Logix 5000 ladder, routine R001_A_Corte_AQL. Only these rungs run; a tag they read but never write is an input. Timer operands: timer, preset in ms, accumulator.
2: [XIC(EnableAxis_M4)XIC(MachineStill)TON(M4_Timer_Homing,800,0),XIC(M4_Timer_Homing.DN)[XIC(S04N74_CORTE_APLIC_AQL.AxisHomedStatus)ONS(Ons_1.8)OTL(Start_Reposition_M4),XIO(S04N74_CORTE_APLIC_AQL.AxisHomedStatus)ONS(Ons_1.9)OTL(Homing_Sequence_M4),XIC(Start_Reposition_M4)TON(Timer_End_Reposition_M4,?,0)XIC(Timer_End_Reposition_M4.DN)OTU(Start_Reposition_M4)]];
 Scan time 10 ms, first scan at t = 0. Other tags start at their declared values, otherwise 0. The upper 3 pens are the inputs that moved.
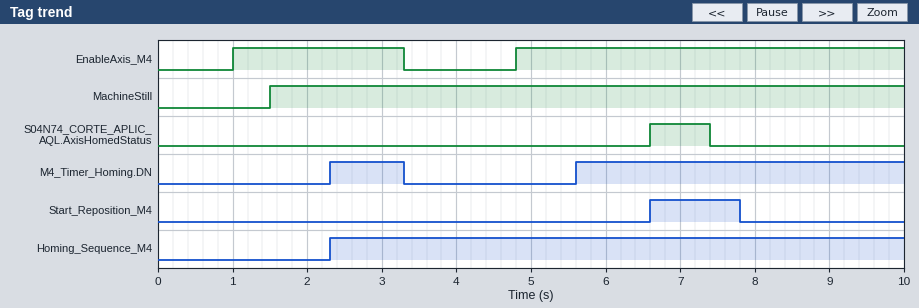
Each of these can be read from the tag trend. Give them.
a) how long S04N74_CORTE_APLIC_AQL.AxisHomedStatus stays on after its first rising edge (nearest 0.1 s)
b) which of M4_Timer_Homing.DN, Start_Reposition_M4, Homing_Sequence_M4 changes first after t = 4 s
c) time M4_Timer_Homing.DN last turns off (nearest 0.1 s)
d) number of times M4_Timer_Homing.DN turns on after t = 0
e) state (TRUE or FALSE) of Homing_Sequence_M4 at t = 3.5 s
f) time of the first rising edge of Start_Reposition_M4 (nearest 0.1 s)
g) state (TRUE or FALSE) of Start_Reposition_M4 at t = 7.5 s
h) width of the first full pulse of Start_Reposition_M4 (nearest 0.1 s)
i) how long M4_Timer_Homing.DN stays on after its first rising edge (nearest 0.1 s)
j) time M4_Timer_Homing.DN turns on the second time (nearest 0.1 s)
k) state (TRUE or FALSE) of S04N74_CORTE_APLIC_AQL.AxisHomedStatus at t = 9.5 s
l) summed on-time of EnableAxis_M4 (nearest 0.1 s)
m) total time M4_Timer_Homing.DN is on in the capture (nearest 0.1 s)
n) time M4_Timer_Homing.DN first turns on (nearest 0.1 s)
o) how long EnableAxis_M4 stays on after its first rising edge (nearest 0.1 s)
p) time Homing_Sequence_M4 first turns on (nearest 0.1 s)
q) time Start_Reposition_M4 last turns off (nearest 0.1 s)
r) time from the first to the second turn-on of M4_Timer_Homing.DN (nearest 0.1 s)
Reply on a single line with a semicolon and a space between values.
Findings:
0.8 s; M4_Timer_Homing.DN; 3.3 s; 2; TRUE; 6.6 s; TRUE; 1.2 s; 1.0 s; 5.6 s; FALSE; 7.5 s; 5.4 s; 2.3 s; 2.3 s; 2.3 s; 7.8 s; 3.3 s
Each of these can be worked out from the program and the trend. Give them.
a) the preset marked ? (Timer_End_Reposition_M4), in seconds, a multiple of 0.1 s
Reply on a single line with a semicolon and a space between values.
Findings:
1.2 s
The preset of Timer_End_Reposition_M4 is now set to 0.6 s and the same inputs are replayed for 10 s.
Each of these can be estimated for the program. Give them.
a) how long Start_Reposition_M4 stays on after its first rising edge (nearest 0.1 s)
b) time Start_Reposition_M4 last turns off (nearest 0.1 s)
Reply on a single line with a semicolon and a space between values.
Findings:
0.6 s; 7.2 s
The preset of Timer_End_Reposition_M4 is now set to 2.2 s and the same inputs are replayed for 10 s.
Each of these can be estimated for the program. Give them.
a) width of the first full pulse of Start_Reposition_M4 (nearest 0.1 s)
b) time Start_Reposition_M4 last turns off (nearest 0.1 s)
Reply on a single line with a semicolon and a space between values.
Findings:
2.2 s; 8.8 s
